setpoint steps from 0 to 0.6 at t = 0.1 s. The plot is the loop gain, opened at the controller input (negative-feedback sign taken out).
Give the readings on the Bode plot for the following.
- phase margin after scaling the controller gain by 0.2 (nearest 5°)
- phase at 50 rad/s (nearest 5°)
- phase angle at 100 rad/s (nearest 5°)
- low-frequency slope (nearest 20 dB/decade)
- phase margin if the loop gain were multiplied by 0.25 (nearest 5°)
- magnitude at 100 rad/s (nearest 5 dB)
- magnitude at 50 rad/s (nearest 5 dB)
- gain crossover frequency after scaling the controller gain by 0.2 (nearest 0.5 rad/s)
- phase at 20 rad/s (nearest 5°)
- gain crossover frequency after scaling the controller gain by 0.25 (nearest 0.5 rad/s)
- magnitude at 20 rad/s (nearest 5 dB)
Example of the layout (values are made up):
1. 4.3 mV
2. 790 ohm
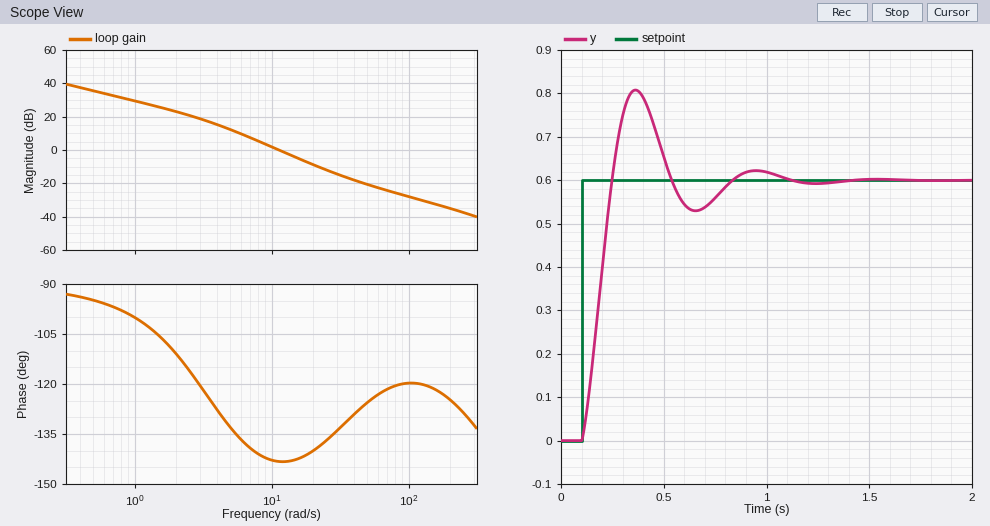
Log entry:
1. 50°
2. -125°
3. -120°
4. -20 dB/decade
5. 45°
6. -30 dB
7. -20 dB
8. 4.5 rad/s
9. -140°
10. 5.0 rad/s
11. -10 dB
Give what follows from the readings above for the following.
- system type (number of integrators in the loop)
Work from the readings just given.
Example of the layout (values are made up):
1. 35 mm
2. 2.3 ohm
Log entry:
1. 1
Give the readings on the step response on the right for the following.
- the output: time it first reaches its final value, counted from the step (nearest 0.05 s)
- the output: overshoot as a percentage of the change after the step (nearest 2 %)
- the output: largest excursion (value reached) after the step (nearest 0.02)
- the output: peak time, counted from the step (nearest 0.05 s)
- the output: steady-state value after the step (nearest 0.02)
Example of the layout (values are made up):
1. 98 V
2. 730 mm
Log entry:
1. 0.15 s
2. 34 %
3. 0.80
4. 0.25 s
5. 0.60
